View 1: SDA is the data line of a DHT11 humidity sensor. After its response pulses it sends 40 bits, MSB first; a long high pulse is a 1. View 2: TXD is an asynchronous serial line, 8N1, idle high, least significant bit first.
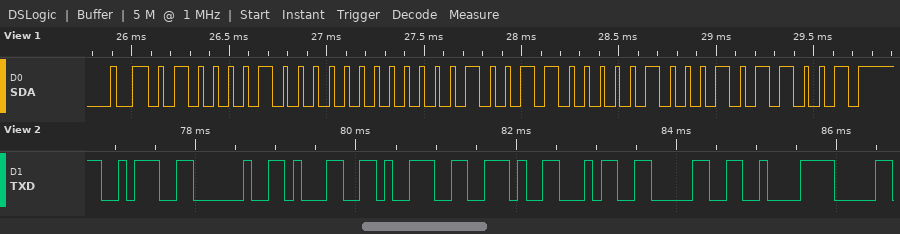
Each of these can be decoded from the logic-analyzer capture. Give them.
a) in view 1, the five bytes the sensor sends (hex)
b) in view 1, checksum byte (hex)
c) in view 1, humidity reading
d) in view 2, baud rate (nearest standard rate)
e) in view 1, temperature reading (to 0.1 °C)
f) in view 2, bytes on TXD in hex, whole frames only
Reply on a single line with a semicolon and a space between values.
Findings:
42 00 13 04 59; 0x59; 66 %; 9600 baud; 19.4 °C; 0x3A 0x20 0x31 0x39 0x2E 0x34 0x30 0xC2
